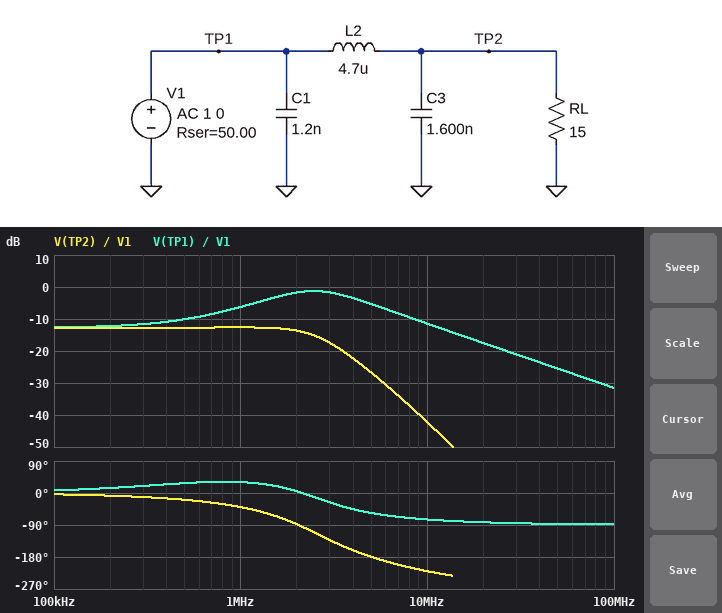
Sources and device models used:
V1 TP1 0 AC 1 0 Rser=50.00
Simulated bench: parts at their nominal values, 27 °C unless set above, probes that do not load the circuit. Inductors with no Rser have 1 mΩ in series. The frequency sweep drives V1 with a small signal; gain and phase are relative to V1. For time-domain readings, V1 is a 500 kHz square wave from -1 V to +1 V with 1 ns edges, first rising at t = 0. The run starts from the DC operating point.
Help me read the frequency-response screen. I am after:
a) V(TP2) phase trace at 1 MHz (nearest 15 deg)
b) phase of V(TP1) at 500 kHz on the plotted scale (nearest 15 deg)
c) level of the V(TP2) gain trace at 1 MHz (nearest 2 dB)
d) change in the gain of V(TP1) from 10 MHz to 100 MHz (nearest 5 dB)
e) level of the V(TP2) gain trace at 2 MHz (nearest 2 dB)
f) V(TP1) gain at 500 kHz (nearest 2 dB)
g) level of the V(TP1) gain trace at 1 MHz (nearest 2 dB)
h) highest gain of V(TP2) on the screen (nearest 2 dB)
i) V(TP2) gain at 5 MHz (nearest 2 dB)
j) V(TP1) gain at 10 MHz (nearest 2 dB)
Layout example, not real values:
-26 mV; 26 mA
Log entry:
-45 deg; 30 deg; -12 dB; -20 dB; -14 dB; -10 dB; -6 dB; -12 dB; -26 dB; -12 dB
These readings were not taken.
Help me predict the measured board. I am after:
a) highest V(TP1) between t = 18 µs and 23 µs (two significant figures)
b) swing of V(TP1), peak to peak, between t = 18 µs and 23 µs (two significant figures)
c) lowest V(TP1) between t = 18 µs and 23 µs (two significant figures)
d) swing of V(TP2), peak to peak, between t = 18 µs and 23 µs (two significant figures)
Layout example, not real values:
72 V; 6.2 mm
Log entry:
1.0 V; 2.0 V; -1.0 V; 530 mV
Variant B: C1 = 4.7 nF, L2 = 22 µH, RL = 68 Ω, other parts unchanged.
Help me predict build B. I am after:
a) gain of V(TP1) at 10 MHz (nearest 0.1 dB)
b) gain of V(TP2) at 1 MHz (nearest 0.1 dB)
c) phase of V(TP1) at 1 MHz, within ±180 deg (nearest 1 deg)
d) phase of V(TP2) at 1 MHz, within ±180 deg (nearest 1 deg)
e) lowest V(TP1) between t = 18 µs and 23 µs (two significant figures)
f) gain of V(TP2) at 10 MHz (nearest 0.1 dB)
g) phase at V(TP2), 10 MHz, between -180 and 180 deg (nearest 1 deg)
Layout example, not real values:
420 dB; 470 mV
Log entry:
-23.4 dB; -10.4 dB; -43 deg; -144 deg; -750 mV; -66.3 dB; 102 deg
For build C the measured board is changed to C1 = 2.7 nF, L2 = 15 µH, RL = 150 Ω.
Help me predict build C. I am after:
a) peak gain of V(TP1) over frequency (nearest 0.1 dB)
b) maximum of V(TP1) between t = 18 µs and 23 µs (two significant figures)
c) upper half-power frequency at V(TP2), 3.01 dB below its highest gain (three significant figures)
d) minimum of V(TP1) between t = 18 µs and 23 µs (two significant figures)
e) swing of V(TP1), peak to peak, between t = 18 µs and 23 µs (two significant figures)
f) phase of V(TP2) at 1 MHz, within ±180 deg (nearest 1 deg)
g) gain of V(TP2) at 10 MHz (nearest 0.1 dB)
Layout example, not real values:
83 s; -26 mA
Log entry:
-2.5 dB; 800 mV; 1.40 MHz; -800 mV; 1.6 V; -97 deg; -58.0 dB
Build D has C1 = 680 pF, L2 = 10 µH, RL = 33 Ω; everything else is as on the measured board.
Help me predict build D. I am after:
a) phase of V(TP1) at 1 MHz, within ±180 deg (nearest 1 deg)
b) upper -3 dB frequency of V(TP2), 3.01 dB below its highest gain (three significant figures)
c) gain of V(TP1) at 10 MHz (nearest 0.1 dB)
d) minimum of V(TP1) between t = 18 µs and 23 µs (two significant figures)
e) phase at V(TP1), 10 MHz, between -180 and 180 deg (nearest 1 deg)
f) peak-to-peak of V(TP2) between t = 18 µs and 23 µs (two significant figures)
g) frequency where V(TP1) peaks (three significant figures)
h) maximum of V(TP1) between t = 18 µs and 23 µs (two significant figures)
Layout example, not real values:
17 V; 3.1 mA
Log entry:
20 deg; 1.55 MHz; -7.2 dB; -1.2 V; -64 deg; 800 mV; 2.47 MHz; 1.2 V
